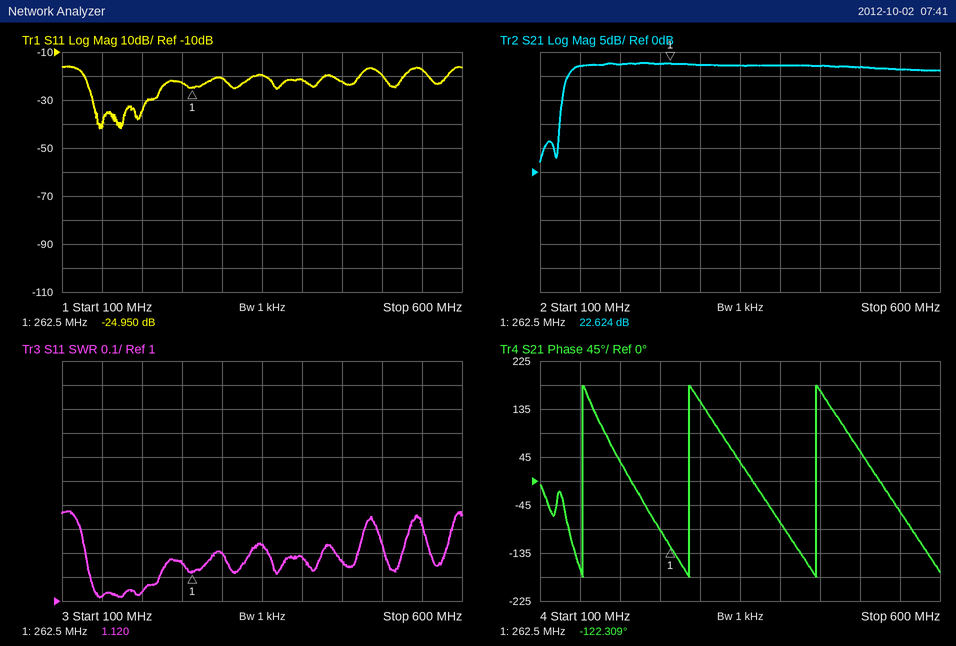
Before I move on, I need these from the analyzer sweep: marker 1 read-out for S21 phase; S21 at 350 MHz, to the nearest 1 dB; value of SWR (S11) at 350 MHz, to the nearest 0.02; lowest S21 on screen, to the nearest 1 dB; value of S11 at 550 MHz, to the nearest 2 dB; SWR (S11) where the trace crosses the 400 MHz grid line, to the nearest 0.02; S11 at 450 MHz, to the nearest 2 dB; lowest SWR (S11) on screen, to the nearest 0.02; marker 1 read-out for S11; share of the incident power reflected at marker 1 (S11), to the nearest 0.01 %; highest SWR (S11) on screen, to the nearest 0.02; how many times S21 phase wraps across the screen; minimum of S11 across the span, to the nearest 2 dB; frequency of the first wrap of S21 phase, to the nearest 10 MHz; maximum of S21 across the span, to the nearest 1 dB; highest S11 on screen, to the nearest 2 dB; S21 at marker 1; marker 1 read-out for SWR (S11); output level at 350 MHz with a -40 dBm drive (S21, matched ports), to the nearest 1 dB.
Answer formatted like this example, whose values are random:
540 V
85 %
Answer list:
-122.309°
22 dB
1.24
2 dB
-18 dB
1.18
-22 dB
1.02
-24.950 dB
0.32 %
1.38
3
-42 dB
150 MHz
23 dB
-16 dB
22.624 dB
1.120
-18 dBm
